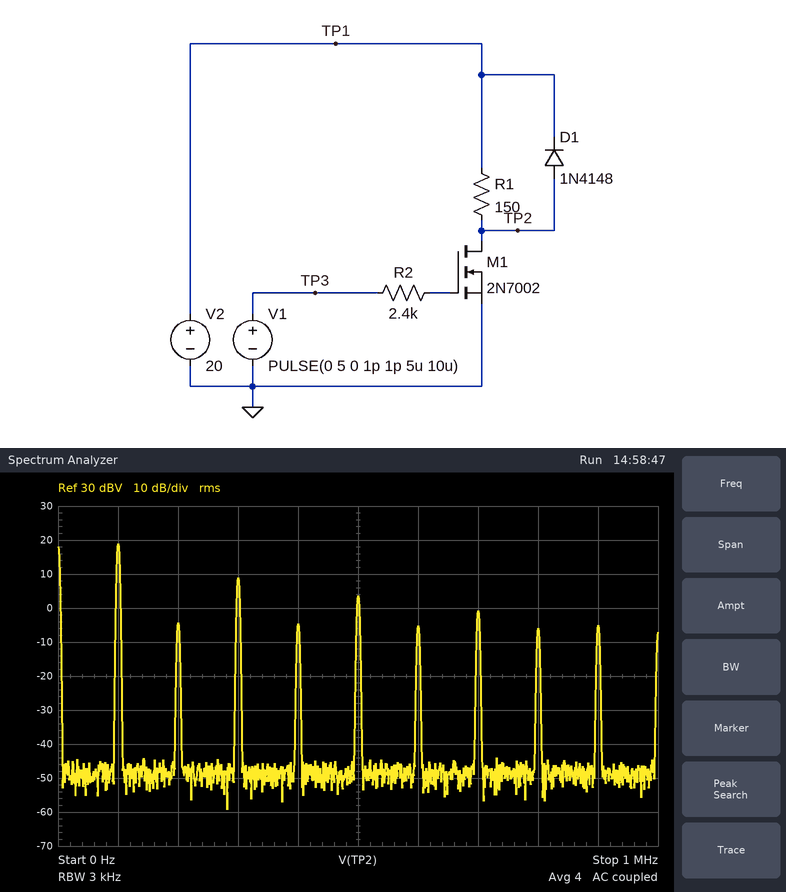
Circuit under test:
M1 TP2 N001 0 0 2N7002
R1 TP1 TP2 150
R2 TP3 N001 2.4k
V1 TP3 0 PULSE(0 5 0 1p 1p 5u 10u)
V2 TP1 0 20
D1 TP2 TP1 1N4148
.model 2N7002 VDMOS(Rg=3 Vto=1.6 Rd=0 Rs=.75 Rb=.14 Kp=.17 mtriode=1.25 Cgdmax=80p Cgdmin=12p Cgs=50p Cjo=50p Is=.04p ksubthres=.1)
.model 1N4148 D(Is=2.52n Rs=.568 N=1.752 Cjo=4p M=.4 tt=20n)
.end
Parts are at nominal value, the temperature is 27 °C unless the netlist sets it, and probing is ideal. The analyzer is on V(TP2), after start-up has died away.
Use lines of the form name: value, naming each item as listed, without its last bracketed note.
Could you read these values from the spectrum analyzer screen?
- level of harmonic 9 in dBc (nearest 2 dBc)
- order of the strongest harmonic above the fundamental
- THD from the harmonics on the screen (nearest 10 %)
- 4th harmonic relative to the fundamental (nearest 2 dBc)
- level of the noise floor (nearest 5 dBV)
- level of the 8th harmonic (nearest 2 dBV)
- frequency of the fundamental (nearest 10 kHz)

level of harmonic 9 in dBc: -24 dBc
order of the strongest harmonic above the fundamental: 3
THD from the harmonics on the screen: 40 %
4th harmonic relative to the fundamental: -24 dBc
level of the noise floor: -50 dBV
level of the 8th harmonic: -6 dBV
frequency of the fundamental: 100 kHz
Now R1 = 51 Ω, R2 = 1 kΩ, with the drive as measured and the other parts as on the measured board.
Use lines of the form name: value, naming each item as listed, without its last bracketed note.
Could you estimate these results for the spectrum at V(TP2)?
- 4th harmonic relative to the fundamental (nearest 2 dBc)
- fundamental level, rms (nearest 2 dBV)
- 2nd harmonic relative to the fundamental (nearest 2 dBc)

4th harmonic relative to the fundamental: -46 dBc
fundamental level, rms: 18 dBV
2nd harmonic relative to the fundamental: -46 dBc
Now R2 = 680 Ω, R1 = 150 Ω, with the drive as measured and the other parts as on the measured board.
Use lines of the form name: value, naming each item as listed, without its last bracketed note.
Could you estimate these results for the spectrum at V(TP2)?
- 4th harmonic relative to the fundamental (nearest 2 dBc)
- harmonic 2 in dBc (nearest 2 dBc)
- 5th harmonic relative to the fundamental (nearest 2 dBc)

4th harmonic relative to the fundamental: -34 dBc
harmonic 2 in dBc: -34 dBc
5th harmonic relative to the fundamental: -14 dBc
